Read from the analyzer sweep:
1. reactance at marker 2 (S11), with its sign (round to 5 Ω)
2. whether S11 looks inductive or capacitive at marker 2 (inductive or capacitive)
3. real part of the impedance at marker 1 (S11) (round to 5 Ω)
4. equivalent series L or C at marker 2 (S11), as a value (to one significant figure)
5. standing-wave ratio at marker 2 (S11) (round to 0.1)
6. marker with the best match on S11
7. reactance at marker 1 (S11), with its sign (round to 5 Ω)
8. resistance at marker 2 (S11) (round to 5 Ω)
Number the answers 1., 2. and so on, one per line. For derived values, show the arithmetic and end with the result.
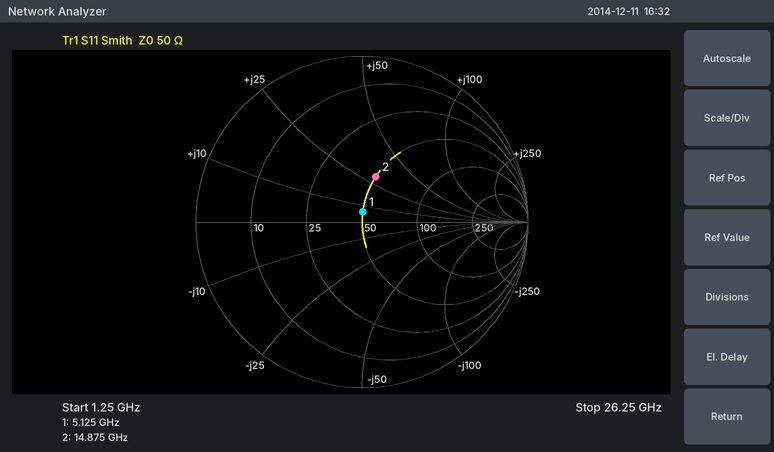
1. +30 Ω
2. inductive
3. 50 Ω
4. L = 30 Ω/(2π × 14.875 GHz) ≈ 321 pH, so 300 pH to one significant figure
5. 1.8
6. marker 1
7. +5 Ω
8. 50 Ω
